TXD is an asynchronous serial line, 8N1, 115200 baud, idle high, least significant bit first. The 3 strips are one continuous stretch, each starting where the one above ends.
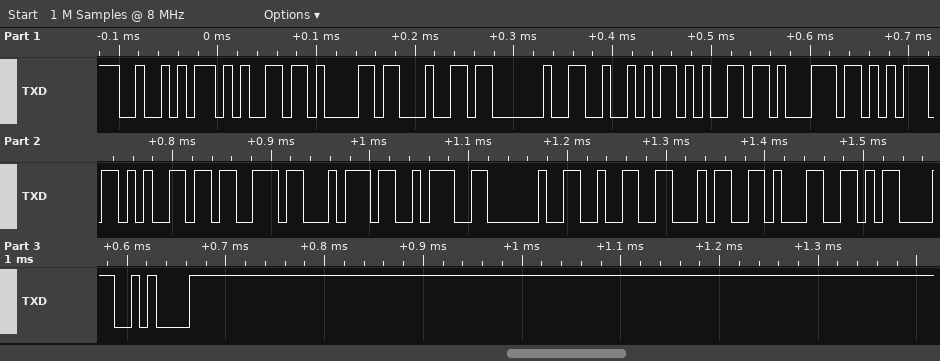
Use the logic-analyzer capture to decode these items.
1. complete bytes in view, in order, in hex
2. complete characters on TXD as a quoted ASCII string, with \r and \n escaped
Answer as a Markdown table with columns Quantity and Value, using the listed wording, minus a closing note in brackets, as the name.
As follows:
| Quantity | Value |
|---|---|
| complete bytes in view, in order, in hex | 52 65 61 64 20 52 65 71 75 65 73 74 3A 20 32 34 31 0D 0A |
| complete characters on TXD as a quoted ASCII string, with \r and \n escaped | "Read Request: 241\r\n" |
